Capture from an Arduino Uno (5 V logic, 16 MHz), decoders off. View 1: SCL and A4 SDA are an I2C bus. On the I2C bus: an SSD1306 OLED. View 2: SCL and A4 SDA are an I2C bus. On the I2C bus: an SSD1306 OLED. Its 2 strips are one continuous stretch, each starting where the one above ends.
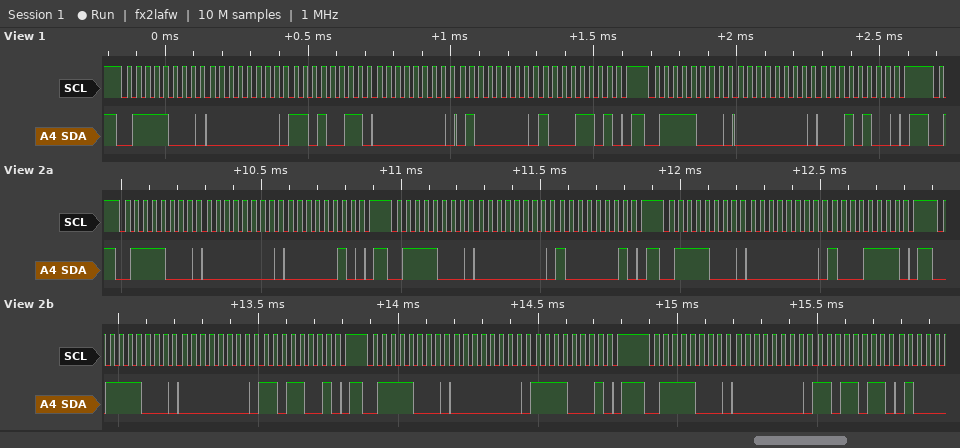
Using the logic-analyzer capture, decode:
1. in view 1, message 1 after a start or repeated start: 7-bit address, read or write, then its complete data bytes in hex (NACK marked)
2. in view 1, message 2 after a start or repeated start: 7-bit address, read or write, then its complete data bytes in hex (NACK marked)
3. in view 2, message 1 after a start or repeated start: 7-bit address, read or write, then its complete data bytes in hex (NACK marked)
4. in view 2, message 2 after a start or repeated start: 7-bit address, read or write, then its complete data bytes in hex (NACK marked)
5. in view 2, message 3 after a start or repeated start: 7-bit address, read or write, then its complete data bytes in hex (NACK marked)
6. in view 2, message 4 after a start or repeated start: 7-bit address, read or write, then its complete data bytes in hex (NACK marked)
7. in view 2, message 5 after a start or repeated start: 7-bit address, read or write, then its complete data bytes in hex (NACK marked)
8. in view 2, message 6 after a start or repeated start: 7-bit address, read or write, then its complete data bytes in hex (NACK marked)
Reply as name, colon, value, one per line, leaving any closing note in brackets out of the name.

in view 1, message 1 after a start or repeated start: 7-bit address, read or write, then its complete data bytes in hex: 0x3C write: 00 D3 00 40 8D
in view 1, message 2 after a start or repeated start: 7-bit address, read or write, then its complete data bytes in hex: 0x3C write: 00 14
in view 2, message 1 after a start or repeated start: 7-bit address, read or write, then its complete data bytes in hex: 0x3C write: 00 02
in view 2, message 2 after a start or repeated start: 7-bit address, read or write, then its complete data bytes in hex: 0x3C write: 00 81
in view 2, message 3 after a start or repeated start: 7-bit address, read or write, then its complete data bytes in hex: 0x3C write: 00 8F
in view 2, message 4 after a start or repeated start: 7-bit address, read or write, then its complete data bytes in hex: 0x3C write: 00 D9
in view 2, message 5 after a start or repeated start: 7-bit address, read or write, then its complete data bytes in hex: 0x3C write: 00 F1
in view 2, message 6 after a start or repeated start: 7-bit address, read or write, then its complete data bytes in hex: 0x3C write: 00 DB
